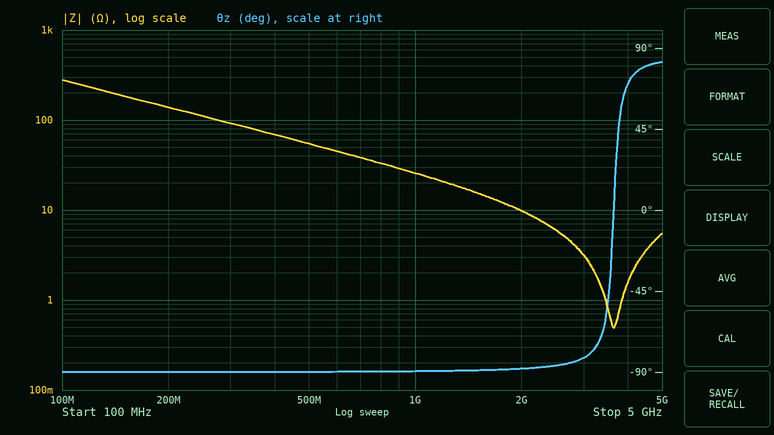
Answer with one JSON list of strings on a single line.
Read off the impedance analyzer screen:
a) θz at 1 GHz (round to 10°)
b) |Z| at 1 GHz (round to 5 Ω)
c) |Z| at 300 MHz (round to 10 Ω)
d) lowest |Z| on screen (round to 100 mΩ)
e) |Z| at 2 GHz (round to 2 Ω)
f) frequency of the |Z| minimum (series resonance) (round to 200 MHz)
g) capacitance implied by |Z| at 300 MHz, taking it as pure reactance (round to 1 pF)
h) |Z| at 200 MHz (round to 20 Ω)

["-90°", "25 Ω", "90 Ω", "500 mΩ", "10 Ω", "3.6 GHz", "6 pF", "140 Ω"]
